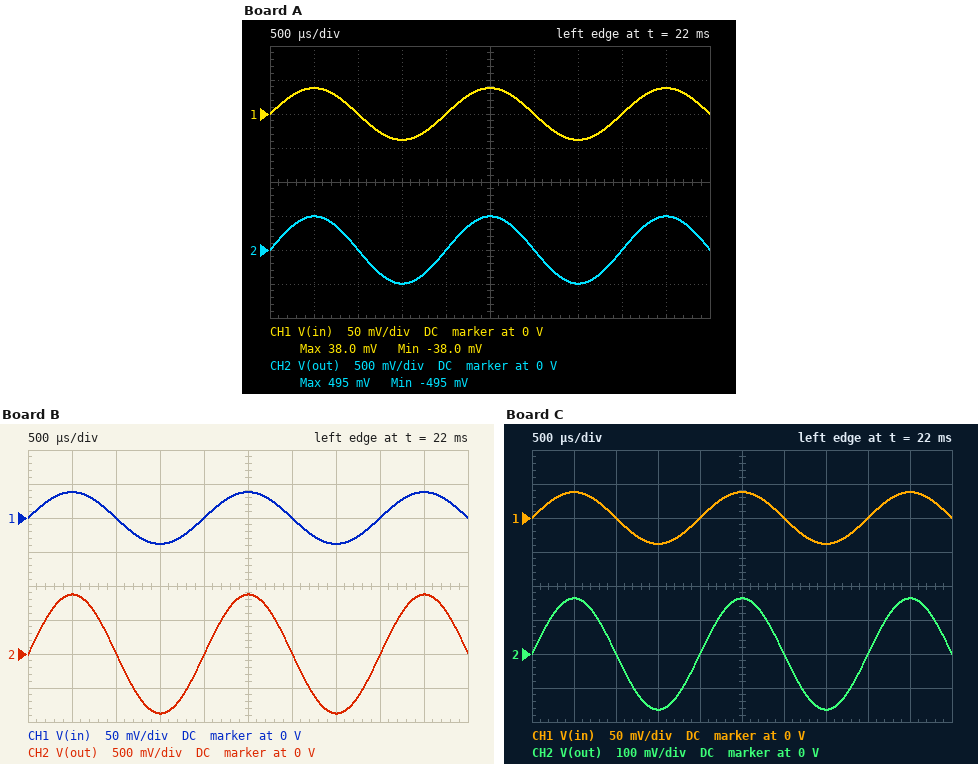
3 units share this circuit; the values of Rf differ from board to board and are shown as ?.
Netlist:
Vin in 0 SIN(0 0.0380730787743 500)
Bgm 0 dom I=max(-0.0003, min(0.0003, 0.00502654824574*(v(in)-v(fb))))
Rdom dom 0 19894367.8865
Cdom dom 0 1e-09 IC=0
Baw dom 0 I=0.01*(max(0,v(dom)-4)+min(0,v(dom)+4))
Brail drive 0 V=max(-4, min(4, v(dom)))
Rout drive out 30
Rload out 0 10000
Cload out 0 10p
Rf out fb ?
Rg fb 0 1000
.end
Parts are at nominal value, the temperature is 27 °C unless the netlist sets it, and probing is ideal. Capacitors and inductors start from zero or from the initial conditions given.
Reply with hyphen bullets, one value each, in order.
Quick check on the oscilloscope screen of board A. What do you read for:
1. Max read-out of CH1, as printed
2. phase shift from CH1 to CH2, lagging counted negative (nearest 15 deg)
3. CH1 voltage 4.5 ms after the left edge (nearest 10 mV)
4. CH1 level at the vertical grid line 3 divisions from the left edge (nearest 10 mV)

- 38.0 mV
- 0 deg
- 40 mV
- -40 mV
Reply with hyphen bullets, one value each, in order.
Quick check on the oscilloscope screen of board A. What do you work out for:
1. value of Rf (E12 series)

- 12 kΩ
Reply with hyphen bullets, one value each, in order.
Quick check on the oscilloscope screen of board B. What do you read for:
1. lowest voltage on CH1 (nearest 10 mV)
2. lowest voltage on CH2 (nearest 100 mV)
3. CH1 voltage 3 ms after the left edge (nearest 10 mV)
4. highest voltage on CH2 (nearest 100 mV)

- -40 mV
- -900 mV
- 0 V
- 900 mV
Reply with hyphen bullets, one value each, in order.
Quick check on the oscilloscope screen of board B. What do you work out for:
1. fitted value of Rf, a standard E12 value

- 22 kΩ
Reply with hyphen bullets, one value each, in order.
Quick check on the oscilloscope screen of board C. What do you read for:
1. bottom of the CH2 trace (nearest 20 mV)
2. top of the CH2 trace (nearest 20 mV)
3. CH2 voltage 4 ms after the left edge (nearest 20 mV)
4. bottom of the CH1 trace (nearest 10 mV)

- -160 mV
- 160 mV
- 0 V
- -40 mV
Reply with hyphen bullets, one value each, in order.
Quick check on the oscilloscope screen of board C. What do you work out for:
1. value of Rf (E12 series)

- 3.3 kΩ
